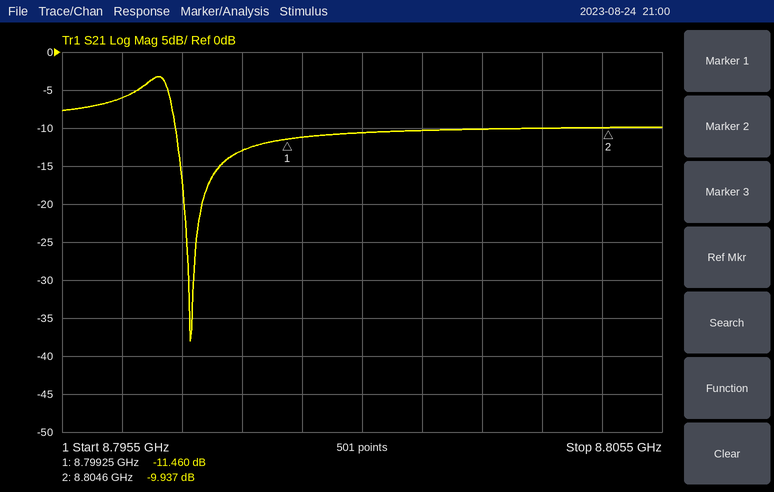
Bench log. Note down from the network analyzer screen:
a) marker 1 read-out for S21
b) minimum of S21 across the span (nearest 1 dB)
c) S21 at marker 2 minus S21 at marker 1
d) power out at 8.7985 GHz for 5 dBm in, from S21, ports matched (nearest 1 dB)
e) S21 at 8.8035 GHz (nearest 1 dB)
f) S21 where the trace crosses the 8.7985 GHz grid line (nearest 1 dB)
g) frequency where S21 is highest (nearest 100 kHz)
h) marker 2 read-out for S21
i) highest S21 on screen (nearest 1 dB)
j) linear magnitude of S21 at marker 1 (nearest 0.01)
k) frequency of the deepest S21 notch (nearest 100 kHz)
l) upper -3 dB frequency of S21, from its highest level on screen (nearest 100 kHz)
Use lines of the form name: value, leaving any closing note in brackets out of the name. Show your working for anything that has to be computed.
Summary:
marker 1 read-out for S21: -11.460 dB
minimum of S21 across the span: -38 dB
S21 at marker 2 minus S21 at marker 1: -9.937 − (-11.46) = 1.523 dB
power out at 8.7985 GHz for 5 dBm in, from S21, ports matched: 5 dBm + (-13 dB) = -8 dBm
S21 at 8.8035 GHz: -10 dB
S21 where the trace crosses the 8.7985 GHz grid line: -13 dB
frequency where S21 is highest: 8.7971 GHz
marker 2 read-out for S21: -9.937 dB
highest S21 on screen: -3 dB
linear magnitude of S21 at marker 1: 10^(-11.46/20) ≈ 0.27
frequency of the deepest S21 notch: 8.7976 GHz
upper -3 dB frequency of S21, from its highest level on screen: 8.7973 GHz
